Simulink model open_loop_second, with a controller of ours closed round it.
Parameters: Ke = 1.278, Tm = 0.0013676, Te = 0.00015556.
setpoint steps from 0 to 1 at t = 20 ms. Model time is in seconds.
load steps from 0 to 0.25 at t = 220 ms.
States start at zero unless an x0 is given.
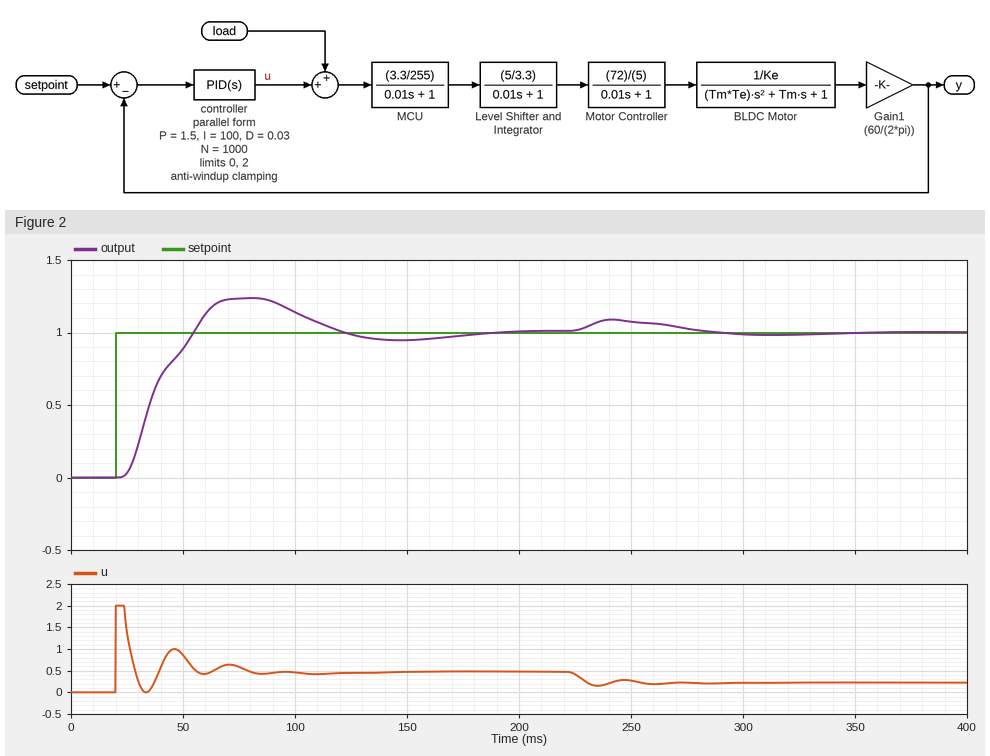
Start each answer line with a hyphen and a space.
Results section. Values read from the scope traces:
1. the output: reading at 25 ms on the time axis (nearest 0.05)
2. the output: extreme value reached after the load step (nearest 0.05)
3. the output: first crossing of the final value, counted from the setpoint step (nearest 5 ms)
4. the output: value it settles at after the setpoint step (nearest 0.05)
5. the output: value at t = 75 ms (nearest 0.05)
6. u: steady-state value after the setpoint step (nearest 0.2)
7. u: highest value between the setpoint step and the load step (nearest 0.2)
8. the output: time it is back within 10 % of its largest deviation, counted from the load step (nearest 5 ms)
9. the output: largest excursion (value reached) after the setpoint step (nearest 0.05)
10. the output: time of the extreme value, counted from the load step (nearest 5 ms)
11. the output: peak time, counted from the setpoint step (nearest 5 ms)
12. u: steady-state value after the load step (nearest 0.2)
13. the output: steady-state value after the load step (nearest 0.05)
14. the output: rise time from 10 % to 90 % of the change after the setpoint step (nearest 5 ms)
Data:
- 0.05
- 1.10
- 35 ms
- 1.00
- 1.25
- 0.4
- 2.0
- 120 ms
- 1.25
- 20 ms
- 60 ms
- 0.2
- 1.00
- 25 ms
